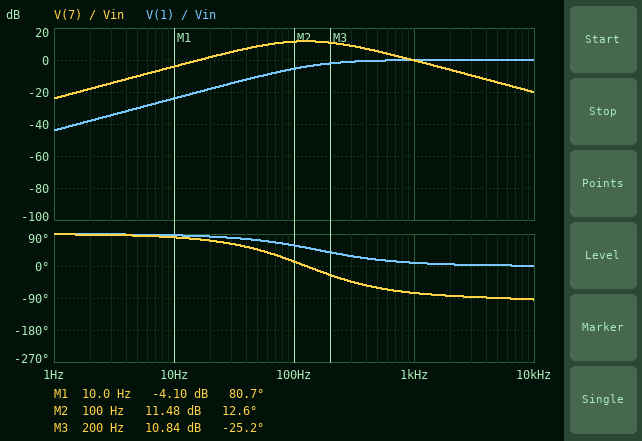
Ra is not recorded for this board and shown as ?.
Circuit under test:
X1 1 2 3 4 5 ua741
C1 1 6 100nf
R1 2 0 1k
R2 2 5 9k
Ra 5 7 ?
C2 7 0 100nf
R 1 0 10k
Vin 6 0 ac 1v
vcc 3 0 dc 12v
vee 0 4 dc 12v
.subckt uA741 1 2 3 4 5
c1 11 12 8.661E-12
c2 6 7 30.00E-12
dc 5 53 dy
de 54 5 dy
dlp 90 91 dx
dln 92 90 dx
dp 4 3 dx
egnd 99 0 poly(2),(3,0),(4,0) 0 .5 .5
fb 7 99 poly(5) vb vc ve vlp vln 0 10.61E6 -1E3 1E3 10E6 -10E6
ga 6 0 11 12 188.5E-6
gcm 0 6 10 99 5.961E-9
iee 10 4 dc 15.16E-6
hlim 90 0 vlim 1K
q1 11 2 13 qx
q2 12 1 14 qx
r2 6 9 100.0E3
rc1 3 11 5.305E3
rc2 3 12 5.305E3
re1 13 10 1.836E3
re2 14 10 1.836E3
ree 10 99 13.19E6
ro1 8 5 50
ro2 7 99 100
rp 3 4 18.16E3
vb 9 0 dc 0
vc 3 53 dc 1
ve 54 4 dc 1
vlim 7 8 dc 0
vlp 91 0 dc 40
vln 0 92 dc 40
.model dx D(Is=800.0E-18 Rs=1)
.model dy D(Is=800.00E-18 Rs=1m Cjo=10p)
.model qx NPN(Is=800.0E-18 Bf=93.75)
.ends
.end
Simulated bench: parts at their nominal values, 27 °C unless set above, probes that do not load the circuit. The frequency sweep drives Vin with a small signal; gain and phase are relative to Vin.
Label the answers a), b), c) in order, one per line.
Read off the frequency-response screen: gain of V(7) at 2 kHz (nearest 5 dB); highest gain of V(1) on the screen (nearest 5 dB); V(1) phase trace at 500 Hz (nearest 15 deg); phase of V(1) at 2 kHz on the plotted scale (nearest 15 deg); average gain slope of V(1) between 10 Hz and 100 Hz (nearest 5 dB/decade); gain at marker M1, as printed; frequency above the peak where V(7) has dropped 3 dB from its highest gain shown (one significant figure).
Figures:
a) -5 dB
b) 0 dB
c) 15 deg
d) 0 deg
e) 20 dB/decade
f) -4.10 dB
g) 300 Hz
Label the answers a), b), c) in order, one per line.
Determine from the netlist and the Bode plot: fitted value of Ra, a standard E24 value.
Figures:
a) 16 kΩ
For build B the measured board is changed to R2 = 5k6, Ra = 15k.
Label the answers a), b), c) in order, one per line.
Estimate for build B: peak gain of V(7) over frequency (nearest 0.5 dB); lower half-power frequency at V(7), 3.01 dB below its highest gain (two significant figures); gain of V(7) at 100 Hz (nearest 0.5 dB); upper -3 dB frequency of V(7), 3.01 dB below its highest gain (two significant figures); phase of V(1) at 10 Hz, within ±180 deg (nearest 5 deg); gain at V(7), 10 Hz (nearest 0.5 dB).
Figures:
a) 8.5 dB
b) 53 Hz
c) 8.0 dB
d) 320 Hz
e) 85 deg
f) -7.5 dB
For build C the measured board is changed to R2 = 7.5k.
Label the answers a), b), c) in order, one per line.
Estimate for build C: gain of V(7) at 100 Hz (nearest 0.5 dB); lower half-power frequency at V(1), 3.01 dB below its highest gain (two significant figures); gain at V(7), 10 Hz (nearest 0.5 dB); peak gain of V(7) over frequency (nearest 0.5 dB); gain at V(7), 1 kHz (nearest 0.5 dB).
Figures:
a) 10.0 dB
b) 160 Hz
c) -5.5 dB
d) 10.5 dB
e) -1.5 dB
